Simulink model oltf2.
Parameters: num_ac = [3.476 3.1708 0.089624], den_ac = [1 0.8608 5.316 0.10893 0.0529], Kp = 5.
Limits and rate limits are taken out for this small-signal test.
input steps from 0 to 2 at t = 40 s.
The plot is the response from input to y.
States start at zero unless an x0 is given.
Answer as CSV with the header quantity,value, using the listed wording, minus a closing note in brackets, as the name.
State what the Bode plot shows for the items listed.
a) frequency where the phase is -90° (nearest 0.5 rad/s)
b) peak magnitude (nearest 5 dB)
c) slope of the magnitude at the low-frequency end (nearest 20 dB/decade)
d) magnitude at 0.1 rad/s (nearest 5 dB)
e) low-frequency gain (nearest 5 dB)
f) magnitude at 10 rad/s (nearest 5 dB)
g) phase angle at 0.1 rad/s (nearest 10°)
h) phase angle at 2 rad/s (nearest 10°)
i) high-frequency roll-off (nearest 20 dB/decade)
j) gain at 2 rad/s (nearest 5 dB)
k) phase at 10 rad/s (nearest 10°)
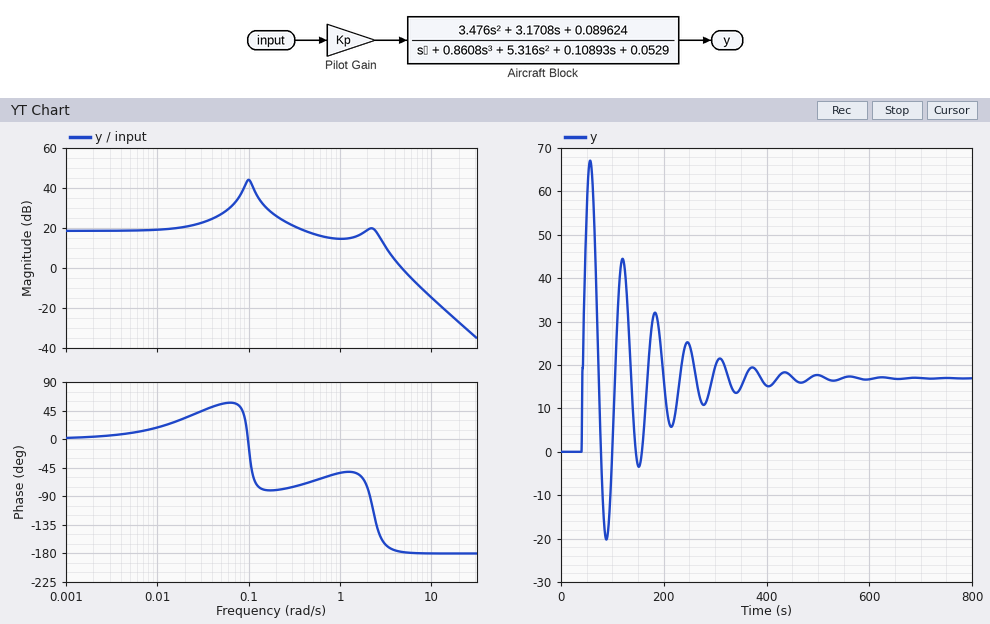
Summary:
quantity,value
frequency where the phase is -90°,2.0 rad/s
peak magnitude,45 dB
slope of the magnitude at the low-frequency end,0 dB/decade
magnitude at 0.1 rad/s,45 dB
low-frequency gain,20 dB
magnitude at 10 rad/s,-15 dB
phase angle at 0.1 rad/s,-10°
phase angle at 2 rad/s,-80°
high-frequency roll-off,-40 dB/decade
gain at 2 rad/s,20 dB
phase at 10 rad/s,-180°
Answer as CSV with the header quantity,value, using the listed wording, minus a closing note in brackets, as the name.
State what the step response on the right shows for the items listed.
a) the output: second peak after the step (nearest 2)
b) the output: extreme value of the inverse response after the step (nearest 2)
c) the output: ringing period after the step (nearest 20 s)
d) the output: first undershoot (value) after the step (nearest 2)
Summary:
quantity,value
the output: second peak after the step,44
the output: extreme value of the inverse response after the step,-20
the output: ringing period after the step,60 s
the output: first undershoot (value) after the step,-20
